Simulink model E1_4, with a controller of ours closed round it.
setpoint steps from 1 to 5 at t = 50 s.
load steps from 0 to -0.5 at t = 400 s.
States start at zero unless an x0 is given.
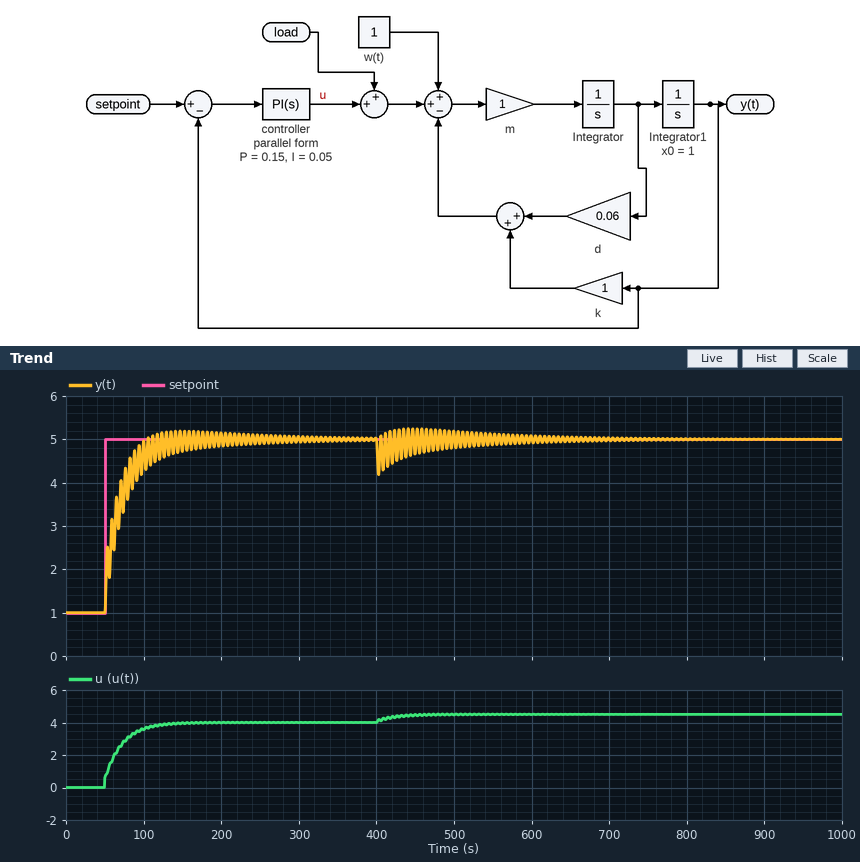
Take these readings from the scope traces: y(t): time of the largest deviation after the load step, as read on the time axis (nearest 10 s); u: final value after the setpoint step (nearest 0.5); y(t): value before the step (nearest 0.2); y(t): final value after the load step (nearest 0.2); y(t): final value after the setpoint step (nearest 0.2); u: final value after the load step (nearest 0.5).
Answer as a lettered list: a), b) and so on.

a) 400 s
b) 4.0
c) 1.0
d) 5.0
e) 5.0
f) 4.5
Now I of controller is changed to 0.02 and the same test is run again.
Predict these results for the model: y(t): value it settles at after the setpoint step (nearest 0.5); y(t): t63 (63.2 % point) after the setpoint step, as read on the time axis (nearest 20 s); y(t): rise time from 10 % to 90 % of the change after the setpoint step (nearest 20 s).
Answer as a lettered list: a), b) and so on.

a) 5.0
b) 100 s
c) 120 s
